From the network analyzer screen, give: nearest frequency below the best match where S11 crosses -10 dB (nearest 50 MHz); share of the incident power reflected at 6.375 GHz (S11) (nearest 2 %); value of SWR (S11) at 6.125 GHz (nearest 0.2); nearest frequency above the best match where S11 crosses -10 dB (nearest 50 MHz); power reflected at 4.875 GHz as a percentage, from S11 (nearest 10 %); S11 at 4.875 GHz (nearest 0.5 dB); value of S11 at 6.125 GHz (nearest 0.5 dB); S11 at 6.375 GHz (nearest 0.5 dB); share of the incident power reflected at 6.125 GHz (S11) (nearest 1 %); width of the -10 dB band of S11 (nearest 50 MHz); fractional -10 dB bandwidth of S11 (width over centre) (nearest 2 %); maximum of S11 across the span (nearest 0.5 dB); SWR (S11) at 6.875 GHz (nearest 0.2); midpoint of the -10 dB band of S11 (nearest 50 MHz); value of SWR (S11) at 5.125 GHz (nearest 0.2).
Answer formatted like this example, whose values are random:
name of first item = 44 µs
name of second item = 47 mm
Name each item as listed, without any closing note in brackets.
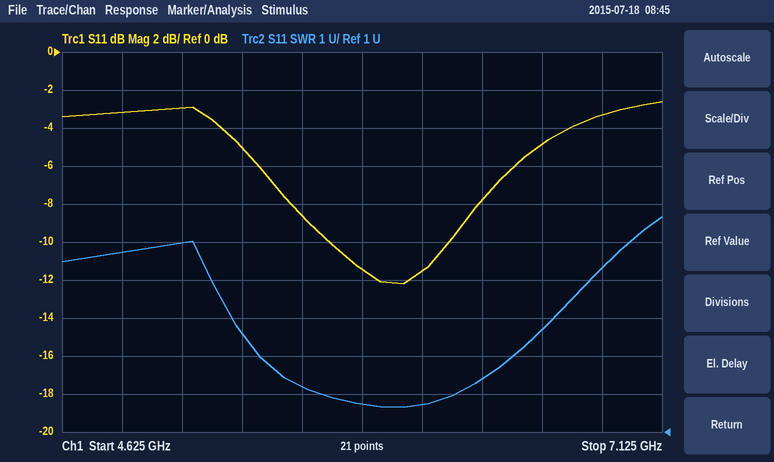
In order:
nearest frequency below the best match where S11 crosses -10 dB = 5.75 GHz
share of the incident power reflected at 6.375 GHz (S11) = 16 %
value of SWR (S11) at 6.125 GHz = 1.8
nearest frequency above the best match where S11 crosses -10 dB = 6.25 GHz
power reflected at 4.875 GHz as a percentage, from S11 = 50 %
S11 at 4.875 GHz = -3.0 dB
value of S11 at 6.125 GHz = -11.5 dB
S11 at 6.375 GHz = -8.0 dB
share of the incident power reflected at 6.125 GHz (S11) = 7 %
width of the -10 dB band of S11 = 500 MHz
fractional -10 dB bandwidth of S11 (width over centre) = 8 %
maximum of S11 across the span = -2.5 dB
SWR (S11) at 6.875 GHz = 5.4
midpoint of the -10 dB band of S11 = 6.00 GHz
value of SWR (S11) at 5.125 GHz = 6.0
